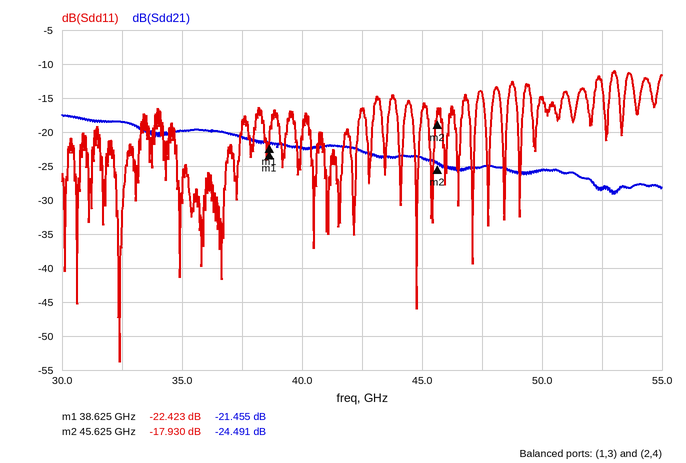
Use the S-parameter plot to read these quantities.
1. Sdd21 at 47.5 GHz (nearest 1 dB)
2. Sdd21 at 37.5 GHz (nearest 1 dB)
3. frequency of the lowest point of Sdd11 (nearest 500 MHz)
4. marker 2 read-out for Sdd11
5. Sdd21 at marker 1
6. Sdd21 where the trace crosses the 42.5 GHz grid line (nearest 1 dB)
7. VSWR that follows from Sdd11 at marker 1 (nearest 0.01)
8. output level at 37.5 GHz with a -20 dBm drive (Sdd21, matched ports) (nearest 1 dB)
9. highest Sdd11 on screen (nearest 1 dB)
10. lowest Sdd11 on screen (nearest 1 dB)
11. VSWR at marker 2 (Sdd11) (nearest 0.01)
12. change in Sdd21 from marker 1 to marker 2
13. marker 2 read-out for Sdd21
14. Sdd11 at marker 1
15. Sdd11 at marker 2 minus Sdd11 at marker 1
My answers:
-25 dB
-21 dB
32.5 GHz
-17.930 dB
-21.455 dB
-23 dB
1.16
-41 dBm
-11 dB
-54 dB
1.29
-3.036 dB
-24.491 dB
-22.423 dB
4.493 dB
